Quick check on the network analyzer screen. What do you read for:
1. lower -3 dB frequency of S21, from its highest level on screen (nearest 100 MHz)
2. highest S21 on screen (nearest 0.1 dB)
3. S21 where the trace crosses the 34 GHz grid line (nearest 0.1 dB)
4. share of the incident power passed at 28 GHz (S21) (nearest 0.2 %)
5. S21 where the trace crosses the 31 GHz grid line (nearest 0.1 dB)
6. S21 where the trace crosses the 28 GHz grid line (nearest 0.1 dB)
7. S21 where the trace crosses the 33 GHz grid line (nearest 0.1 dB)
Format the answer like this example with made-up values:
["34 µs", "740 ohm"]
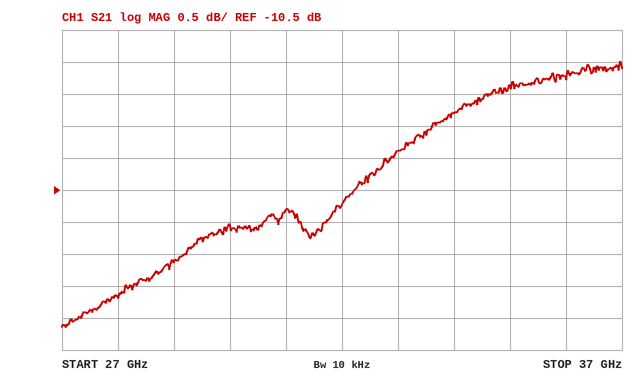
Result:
["29.2 GHz", "-8.5 dB", "-9.3 dB", "6.0 %", "-10.8 dB", "-12.2 dB", "-9.9 dB"]
